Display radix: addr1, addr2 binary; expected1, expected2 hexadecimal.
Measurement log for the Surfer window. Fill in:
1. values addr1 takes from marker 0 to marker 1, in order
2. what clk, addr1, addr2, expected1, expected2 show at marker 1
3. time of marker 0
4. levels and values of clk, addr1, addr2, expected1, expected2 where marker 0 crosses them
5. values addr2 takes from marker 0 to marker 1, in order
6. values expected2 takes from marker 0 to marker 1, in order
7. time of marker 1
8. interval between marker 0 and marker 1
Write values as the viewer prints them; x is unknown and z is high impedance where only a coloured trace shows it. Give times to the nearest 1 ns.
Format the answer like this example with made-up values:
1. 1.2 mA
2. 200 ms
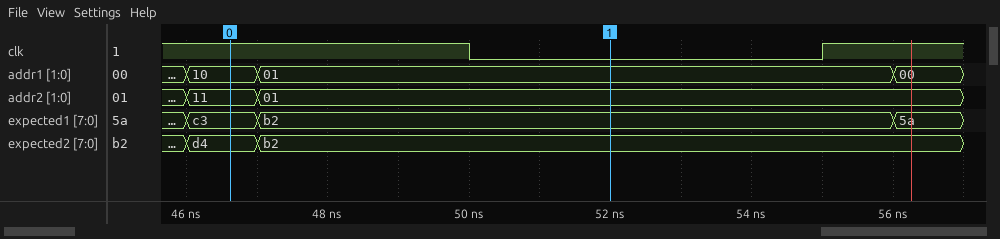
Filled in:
1. 10, 01
2. clk=0, addr1=01, addr2=01, expected1=b2, expected2=b2
3. 47 ns
4. clk=1, addr1=10, addr2=11, expected1=c3, expected2=d4
5. 11, 01
6. d4, b2
7. 52 ns
8. 5 ns
